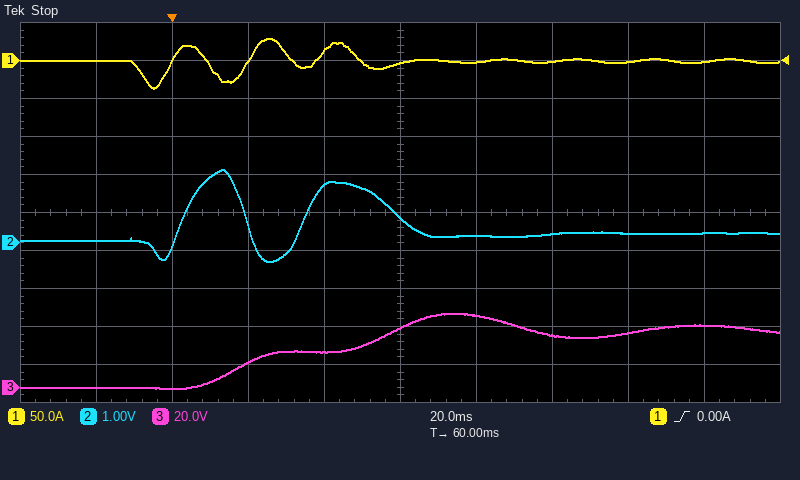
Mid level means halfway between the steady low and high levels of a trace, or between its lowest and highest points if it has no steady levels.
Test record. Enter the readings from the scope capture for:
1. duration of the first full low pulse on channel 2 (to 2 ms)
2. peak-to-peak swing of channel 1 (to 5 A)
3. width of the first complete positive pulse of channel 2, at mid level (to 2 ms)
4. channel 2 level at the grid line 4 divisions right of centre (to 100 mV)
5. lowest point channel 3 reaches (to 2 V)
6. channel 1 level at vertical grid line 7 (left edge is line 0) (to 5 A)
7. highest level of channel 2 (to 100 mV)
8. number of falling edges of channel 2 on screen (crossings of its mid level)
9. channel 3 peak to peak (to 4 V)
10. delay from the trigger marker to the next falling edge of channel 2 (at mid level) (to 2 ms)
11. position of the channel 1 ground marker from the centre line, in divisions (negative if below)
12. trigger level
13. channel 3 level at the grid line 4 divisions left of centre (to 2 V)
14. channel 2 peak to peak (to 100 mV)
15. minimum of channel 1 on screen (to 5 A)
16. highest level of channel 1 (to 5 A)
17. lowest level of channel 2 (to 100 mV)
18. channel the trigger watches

16 ms
65 A
16 ms
300 mV
0 V
0 A
1.9 V
2
40 V
20 ms
+4.0 div
0.00 A
0 V
2.4 V
-35 A
30 A
-500 mV
channel 1
